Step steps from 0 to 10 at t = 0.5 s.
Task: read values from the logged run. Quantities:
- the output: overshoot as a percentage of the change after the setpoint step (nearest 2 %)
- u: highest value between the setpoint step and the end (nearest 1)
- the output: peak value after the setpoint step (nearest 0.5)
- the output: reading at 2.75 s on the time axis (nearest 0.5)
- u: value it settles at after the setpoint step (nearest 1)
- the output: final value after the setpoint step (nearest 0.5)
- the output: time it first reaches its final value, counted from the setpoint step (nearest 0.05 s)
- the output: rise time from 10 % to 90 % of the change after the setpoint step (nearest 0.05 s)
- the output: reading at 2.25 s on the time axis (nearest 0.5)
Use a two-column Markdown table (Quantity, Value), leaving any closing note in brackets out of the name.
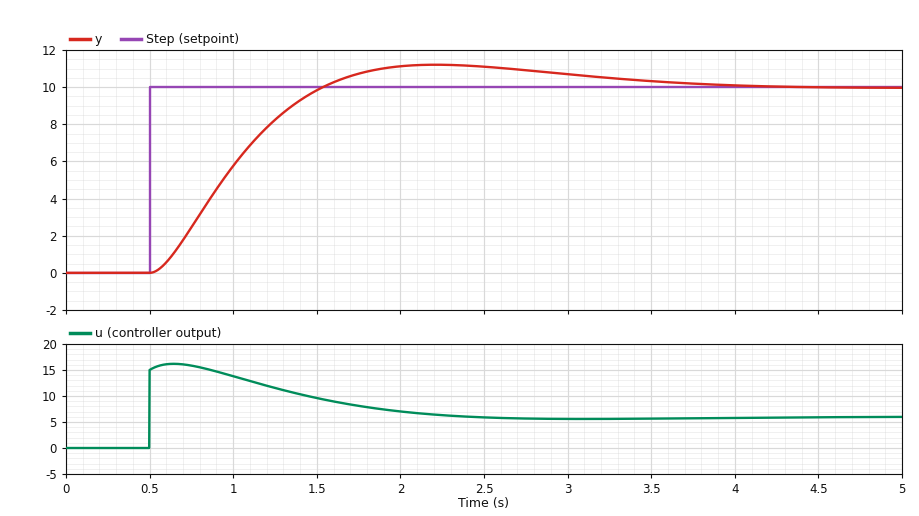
| Quantity | Value |
|---|---|
| the output: overshoot as a percentage of the change after the setpoint step | 12 % |
| u: highest value between the setpoint step and the end | 16 |
| the output: peak value after the setpoint step | 11.0 |
| the output: reading at 2.75 s on the time axis | 11.0 |
| u: value it settles at after the setpoint step | 6 |
| the output: final value after the setpoint step | 10.0 |
| the output: time it first reaches its final value, counted from the setpoint step | 1.05 s |
| the output: rise time from 10 % to 90 % of the change after the setpoint step | 0.70 s |
| the output: reading at 2.25 s on the time axis | 11.0 |
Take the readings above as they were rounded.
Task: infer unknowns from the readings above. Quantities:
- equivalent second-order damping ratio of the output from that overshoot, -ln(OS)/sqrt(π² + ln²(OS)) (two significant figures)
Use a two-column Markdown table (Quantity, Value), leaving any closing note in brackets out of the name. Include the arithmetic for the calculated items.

| Quantity | Value |
|---|---|
| equivalent second-order damping ratio of the output from that overshoot, -ln(OS)/sqrt(π² + ln²(OS)) | ln(0.12) = -2.120; 2.120 / sqrt(9.870 + 4.496) = 0.56 |
